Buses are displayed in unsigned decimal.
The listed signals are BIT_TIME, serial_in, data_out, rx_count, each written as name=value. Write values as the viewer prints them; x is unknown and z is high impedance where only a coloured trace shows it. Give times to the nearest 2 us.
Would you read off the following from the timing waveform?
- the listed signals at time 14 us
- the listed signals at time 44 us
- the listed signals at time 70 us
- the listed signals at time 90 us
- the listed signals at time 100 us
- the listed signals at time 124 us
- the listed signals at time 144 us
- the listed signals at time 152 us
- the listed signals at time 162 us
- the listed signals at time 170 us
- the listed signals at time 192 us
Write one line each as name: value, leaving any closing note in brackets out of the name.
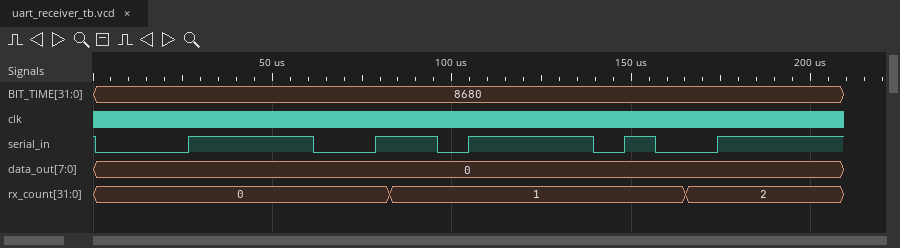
the listed signals at time 14 us: BIT_TIME=8680, serial_in=0, data_out=0, rx_count=0
the listed signals at time 44 us: BIT_TIME=8680, serial_in=1, data_out=0, rx_count=0
the listed signals at time 70 us: BIT_TIME=8680, serial_in=0, data_out=0, rx_count=0
the listed signals at time 90 us: BIT_TIME=8680, serial_in=1, data_out=0, rx_count=1
the listed signals at time 100 us: BIT_TIME=8680, serial_in=0, data_out=0, rx_count=1
the listed signals at time 124 us: BIT_TIME=8680, serial_in=1, data_out=0, rx_count=1
the listed signals at time 144 us: BIT_TIME=8680, serial_in=0, data_out=0, rx_count=1
the listed signals at time 152 us: BIT_TIME=8680, serial_in=1, data_out=0, rx_count=1
the listed signals at time 162 us: BIT_TIME=8680, serial_in=0, data_out=0, rx_count=1
the listed signals at time 170 us: BIT_TIME=8680, serial_in=0, data_out=0, rx_count=2
the listed signals at time 192 us: BIT_TIME=8680, serial_in=1, data_out=0, rx_count=2
